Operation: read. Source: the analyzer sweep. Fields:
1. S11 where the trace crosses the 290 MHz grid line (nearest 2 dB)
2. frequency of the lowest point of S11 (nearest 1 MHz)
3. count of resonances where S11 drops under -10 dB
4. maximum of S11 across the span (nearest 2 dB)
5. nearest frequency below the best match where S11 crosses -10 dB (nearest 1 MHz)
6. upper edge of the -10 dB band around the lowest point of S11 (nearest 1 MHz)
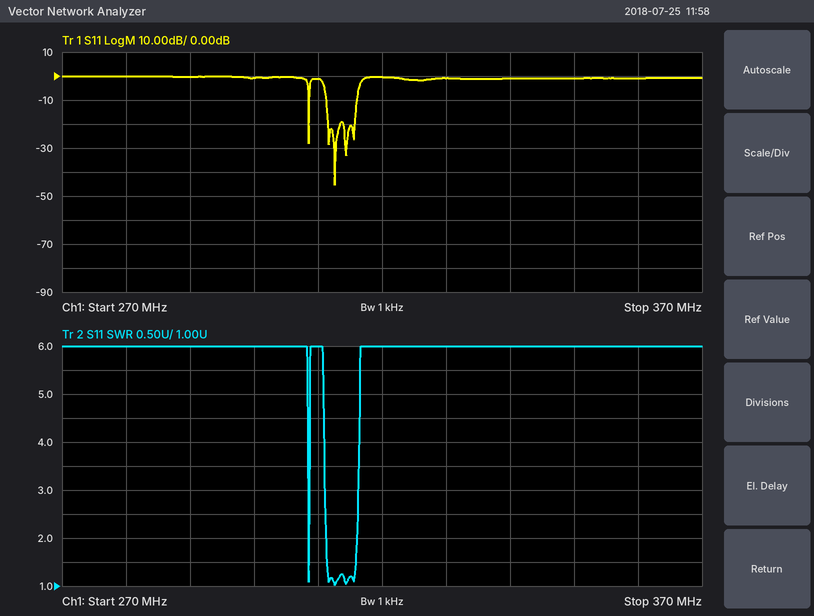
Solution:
0 dB
313 MHz
5
0 dB
311 MHz
316 MHz
